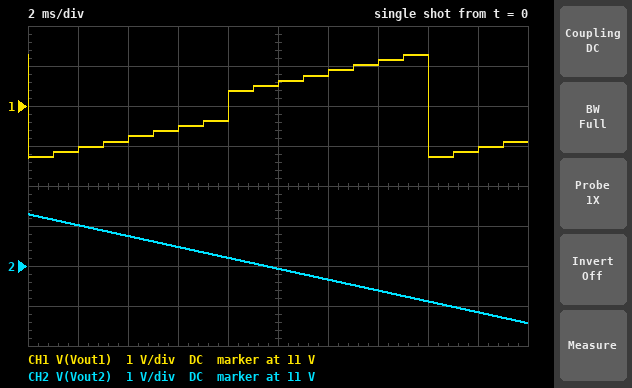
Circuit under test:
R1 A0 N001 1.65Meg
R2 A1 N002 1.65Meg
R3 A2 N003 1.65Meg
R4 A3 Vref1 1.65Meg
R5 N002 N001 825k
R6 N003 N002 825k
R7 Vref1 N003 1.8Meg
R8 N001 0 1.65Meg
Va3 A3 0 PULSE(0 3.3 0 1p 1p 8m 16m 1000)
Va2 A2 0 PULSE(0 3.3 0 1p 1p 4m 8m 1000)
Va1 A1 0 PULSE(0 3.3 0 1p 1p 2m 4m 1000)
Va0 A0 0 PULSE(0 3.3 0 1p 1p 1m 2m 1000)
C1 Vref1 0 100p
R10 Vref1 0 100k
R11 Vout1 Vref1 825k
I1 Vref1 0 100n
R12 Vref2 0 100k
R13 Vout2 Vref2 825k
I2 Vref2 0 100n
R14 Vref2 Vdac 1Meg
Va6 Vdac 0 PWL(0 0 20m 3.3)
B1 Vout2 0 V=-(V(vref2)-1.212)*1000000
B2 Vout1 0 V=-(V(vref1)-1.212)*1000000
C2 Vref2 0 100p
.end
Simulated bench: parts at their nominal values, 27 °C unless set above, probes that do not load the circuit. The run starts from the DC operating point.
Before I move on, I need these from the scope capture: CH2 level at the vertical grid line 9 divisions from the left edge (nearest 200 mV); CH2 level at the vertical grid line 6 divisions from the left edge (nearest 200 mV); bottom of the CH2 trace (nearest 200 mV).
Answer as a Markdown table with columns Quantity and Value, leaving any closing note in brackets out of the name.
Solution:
| Quantity | Value |
|---|---|
| CH2 level at the vertical grid line 9 divisions from the left edge | 9.8 V |
| CH2 level at the vertical grid line 6 divisions from the left edge | 10.6 V |
| bottom of the CH2 trace | 9.6 V |
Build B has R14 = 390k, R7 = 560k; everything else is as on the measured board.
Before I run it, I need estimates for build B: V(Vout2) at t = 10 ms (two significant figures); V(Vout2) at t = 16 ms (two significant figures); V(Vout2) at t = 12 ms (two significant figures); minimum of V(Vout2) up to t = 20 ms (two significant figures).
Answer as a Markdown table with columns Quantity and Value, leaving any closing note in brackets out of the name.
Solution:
| Quantity | Value |
|---|---|
| V(Vout2) at t = 10 ms | 10 V |
| V(Vout2) at t = 16 ms | 8.3 V |
| V(Vout2) at t = 12 ms | 9.7 V |
| minimum of V(Vout2) up to t = 20 ms | 6.9 V |
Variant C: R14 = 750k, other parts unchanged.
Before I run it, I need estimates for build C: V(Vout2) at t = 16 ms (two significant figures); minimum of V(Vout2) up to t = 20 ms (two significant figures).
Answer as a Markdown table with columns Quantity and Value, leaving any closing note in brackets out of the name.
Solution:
| Quantity | Value |
|---|---|
| V(Vout2) at t = 16 ms | 9.7 V |
| minimum of V(Vout2) up to t = 20 ms | 9.0 V |
